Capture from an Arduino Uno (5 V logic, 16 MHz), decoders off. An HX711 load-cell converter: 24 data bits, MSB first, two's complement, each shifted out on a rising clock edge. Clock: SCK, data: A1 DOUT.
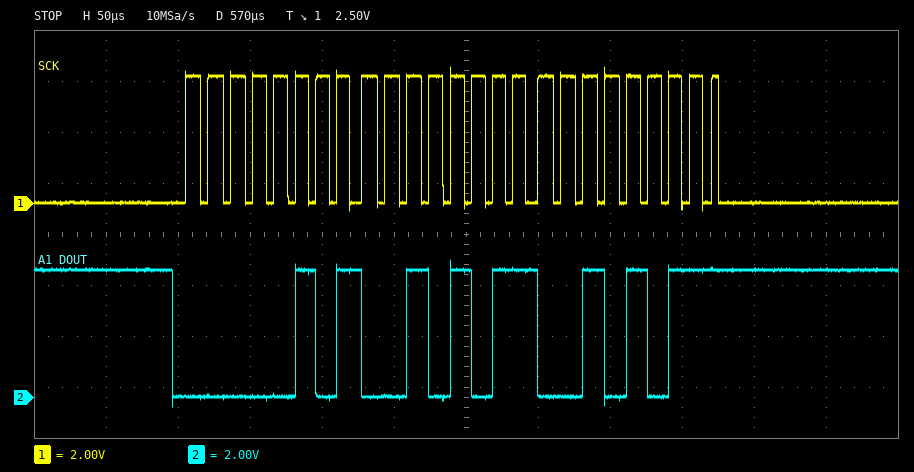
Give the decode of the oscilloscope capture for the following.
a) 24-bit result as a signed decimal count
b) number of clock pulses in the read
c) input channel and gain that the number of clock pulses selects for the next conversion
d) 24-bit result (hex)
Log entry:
338731
25
channel A, gain 128
0x052B2B
